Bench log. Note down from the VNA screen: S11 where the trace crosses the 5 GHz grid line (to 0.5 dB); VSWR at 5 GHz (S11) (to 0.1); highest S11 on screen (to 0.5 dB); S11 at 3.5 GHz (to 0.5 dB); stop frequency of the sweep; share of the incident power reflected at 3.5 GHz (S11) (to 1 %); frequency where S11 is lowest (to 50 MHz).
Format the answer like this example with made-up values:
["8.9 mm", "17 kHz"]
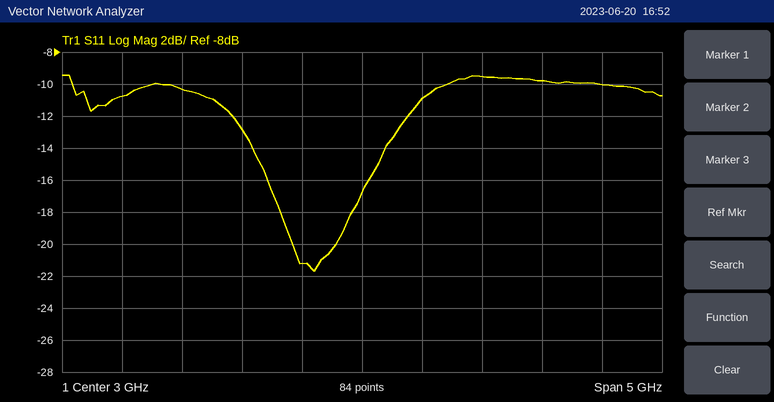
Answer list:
["-10.0 dB", "1.9", "-9.5 dB", "-11.0 dB", "5.5 GHz", "8 %", "2.60 GHz"]
